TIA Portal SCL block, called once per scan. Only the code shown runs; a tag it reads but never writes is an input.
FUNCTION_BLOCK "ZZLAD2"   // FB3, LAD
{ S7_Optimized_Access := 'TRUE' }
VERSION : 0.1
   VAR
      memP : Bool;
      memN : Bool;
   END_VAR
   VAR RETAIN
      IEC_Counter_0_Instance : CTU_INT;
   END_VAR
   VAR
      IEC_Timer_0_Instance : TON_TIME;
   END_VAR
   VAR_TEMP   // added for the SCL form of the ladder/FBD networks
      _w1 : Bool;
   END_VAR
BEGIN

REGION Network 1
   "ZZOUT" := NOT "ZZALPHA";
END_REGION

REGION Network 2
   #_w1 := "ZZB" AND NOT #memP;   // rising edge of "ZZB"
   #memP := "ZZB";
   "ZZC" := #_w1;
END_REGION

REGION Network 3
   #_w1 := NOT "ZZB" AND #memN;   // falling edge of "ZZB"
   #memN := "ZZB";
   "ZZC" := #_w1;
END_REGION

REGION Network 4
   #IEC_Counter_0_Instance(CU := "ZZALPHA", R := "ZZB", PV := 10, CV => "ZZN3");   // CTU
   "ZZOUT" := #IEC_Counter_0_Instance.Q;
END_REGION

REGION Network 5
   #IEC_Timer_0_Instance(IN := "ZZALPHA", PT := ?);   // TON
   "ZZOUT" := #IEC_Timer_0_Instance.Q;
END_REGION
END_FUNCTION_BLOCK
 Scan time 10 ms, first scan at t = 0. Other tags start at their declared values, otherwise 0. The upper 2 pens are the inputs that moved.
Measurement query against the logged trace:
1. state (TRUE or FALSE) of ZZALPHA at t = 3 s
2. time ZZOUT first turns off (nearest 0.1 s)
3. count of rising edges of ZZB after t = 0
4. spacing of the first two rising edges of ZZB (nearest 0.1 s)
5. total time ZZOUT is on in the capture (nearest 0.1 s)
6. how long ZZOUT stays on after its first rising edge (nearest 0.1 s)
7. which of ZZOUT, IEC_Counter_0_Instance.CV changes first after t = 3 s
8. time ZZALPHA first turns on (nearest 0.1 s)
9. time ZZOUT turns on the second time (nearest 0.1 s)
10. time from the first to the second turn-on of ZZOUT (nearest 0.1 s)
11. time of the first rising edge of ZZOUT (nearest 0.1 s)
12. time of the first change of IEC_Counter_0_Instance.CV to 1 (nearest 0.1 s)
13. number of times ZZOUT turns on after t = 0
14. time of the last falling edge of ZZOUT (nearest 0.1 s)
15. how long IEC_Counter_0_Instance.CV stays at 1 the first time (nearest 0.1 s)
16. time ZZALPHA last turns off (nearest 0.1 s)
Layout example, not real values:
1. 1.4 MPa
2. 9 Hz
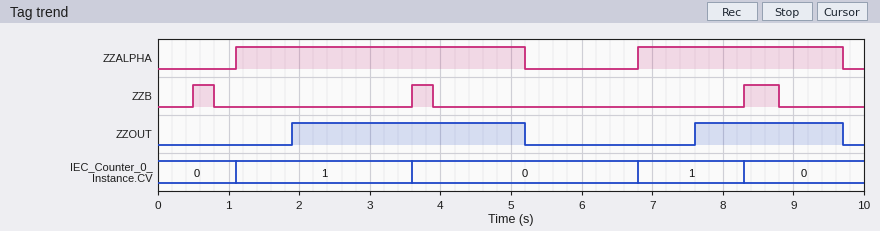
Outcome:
1. TRUE
2. 5.2 s
3. 3
4. 3.1 s
5. 5.4 s
6. 3.3 s
7. IEC_Counter_0_Instance.CV
8. 1.1 s
9. 7.6 s
10. 5.7 s
11. 1.9 s
12. 1.1 s
13. 2
14. 9.7 s
15. 2.5 s
16. 9.7 s
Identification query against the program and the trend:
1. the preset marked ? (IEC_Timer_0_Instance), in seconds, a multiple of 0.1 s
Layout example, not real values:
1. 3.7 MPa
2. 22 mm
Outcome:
1. 0.8 s
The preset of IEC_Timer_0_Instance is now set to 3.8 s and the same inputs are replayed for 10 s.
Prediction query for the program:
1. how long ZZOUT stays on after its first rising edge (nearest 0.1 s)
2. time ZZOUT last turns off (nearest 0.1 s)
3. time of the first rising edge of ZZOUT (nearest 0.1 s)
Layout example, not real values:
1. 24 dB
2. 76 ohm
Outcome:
1. 0.3 s
2. 5.2 s
3. 4.9 s
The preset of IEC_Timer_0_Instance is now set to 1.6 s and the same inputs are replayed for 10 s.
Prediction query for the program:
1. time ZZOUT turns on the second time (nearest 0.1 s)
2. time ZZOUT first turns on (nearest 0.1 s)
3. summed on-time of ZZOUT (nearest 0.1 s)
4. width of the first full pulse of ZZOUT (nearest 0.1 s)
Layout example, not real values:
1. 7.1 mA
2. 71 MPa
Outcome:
1. 8.4 s
2. 2.7 s
3. 3.8 s
4. 2.5 s
